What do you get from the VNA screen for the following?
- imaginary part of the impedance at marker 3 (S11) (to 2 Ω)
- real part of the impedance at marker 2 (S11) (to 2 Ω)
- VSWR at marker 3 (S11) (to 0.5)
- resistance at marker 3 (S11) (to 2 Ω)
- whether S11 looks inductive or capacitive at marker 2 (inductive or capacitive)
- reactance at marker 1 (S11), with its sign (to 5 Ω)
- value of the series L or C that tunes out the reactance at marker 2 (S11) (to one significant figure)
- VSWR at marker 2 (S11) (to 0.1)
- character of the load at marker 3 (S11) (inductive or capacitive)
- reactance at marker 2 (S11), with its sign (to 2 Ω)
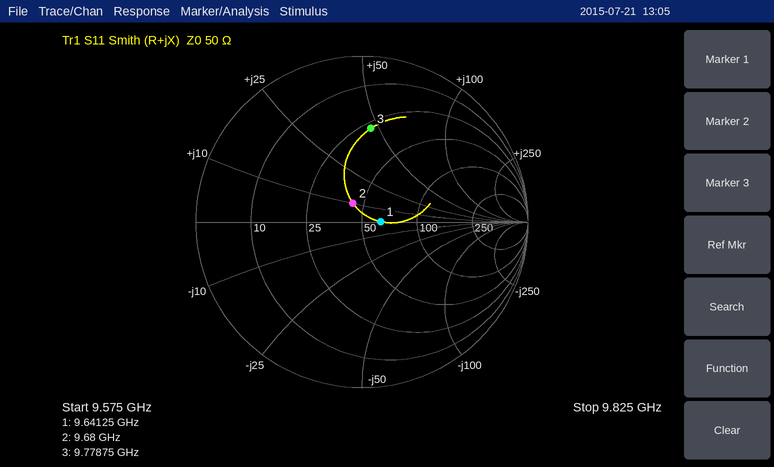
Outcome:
+46 Ω
44 Ω
3.5
28 Ω
inductive
0 Ω
2 pF
1.3
inductive
+10 Ω
